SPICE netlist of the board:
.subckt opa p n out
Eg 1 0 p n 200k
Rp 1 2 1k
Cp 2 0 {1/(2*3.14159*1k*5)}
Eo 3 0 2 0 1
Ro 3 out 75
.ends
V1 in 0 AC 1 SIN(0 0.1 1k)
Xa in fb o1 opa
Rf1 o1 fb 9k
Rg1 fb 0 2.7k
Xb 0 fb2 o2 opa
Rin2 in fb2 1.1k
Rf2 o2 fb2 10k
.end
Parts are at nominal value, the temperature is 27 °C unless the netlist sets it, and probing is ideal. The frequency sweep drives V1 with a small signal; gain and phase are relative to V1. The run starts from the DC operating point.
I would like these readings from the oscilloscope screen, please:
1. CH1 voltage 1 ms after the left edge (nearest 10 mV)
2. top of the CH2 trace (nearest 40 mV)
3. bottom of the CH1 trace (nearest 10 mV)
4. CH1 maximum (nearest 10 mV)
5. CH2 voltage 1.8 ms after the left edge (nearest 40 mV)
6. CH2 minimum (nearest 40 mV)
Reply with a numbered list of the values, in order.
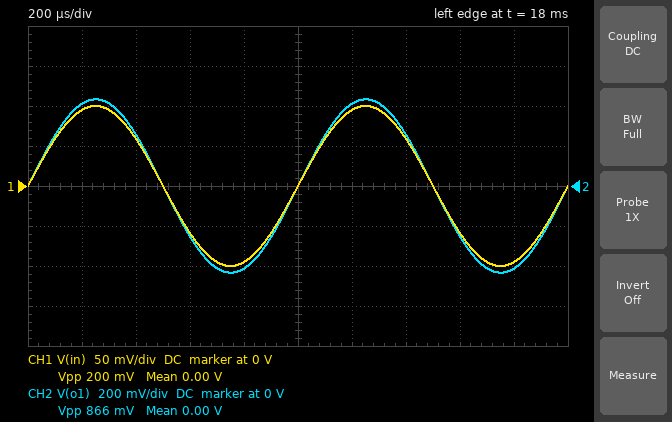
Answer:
1. 0 V
2. 440 mV
3. -100 mV
4. 100 mV
5. -400 mV
6. -440 mV
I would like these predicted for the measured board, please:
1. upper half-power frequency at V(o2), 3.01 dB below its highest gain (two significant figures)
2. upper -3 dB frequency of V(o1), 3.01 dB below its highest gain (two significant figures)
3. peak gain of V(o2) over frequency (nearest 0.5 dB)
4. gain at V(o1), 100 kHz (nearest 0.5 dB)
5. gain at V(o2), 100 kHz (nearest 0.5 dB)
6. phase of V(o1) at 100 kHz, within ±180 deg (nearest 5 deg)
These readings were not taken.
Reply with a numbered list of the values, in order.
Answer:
1. 98 kHz
2. 230 kHz
3. 19.0 dB
4. 12.0 dB
5. 16.0 dB
6. -25 deg
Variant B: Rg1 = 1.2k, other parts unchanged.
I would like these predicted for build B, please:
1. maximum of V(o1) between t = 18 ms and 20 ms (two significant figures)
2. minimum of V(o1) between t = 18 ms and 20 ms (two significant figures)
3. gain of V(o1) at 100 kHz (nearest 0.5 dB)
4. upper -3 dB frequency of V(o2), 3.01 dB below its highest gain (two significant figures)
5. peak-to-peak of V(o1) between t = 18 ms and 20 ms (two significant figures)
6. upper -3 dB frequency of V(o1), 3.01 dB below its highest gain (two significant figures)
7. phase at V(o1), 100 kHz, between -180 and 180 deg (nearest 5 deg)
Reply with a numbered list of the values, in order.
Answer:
1. 850 mV
2. -850 mV
3. 16.0 dB
4. 98 kHz
5. 1.7 V
6. 120 kHz
7. -40 deg
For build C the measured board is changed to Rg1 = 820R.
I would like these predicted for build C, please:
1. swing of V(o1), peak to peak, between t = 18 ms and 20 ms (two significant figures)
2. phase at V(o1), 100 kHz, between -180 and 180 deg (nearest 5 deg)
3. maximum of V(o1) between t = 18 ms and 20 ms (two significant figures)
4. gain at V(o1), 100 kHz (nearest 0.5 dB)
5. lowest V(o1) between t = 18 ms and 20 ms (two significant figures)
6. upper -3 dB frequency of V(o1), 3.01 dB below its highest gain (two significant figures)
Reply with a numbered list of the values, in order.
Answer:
1. 2.4 V
2. -50 deg
3. 1.2 V
4. 17.5 dB
5. -1.2 V
6. 83 kHz
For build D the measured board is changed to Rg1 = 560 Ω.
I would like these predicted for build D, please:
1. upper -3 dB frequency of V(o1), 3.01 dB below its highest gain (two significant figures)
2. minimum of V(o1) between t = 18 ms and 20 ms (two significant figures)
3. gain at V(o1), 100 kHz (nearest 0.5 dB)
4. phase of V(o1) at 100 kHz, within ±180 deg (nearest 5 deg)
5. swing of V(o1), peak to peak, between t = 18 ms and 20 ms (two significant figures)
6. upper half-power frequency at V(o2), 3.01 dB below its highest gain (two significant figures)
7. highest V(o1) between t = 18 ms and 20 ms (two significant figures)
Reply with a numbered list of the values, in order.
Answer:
1. 58 kHz
2. -1.7 V
3. 18.5 dB
4. -60 deg
5. 3.4 V
6. 98 kHz
7. 1.7 V
